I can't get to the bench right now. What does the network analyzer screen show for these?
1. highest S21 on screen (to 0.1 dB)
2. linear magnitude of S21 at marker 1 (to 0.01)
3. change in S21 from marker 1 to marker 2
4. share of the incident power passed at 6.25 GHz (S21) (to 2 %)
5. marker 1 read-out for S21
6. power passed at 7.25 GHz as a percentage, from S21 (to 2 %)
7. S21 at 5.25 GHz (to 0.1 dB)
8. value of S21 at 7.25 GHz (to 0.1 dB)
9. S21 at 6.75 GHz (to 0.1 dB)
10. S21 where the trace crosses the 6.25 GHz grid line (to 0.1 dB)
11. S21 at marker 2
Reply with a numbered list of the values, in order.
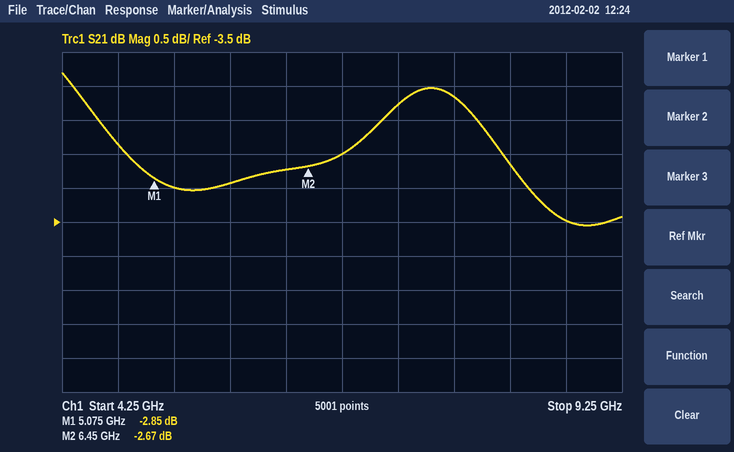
1. -1.3 dB
2. 0.72
3. 0.18 dB
4. 54 %
5. -2.85 dB
6. 66 %
7. -3.0 dB
8. -1.8 dB
9. -2.5 dB
10. -2.7 dB
11. -2.67 dB
